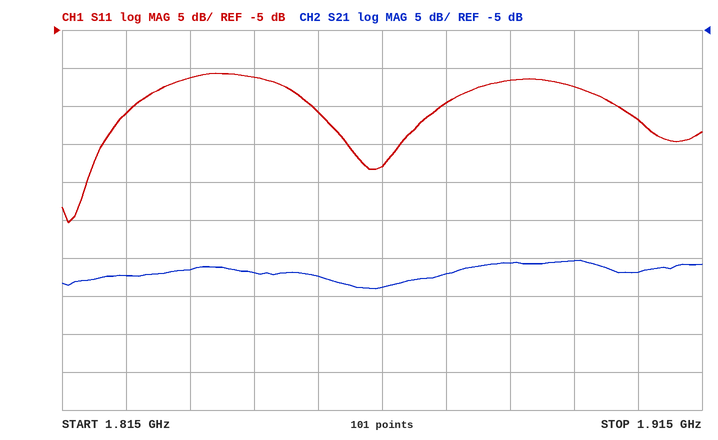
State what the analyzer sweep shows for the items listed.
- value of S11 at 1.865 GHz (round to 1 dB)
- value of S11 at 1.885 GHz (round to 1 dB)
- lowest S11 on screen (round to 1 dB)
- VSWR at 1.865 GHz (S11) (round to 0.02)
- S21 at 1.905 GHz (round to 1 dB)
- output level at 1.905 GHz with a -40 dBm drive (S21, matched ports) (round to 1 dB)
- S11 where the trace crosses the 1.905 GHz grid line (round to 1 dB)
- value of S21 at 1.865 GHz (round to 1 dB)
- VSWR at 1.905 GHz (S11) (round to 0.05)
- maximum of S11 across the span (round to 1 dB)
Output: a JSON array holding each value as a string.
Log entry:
["-23 dB", "-12 dB", "-30 dB", "1.16", "-37 dB", "-77 dBm", "-17 dB", "-39 dB", "1.35", "-11 dB"]
